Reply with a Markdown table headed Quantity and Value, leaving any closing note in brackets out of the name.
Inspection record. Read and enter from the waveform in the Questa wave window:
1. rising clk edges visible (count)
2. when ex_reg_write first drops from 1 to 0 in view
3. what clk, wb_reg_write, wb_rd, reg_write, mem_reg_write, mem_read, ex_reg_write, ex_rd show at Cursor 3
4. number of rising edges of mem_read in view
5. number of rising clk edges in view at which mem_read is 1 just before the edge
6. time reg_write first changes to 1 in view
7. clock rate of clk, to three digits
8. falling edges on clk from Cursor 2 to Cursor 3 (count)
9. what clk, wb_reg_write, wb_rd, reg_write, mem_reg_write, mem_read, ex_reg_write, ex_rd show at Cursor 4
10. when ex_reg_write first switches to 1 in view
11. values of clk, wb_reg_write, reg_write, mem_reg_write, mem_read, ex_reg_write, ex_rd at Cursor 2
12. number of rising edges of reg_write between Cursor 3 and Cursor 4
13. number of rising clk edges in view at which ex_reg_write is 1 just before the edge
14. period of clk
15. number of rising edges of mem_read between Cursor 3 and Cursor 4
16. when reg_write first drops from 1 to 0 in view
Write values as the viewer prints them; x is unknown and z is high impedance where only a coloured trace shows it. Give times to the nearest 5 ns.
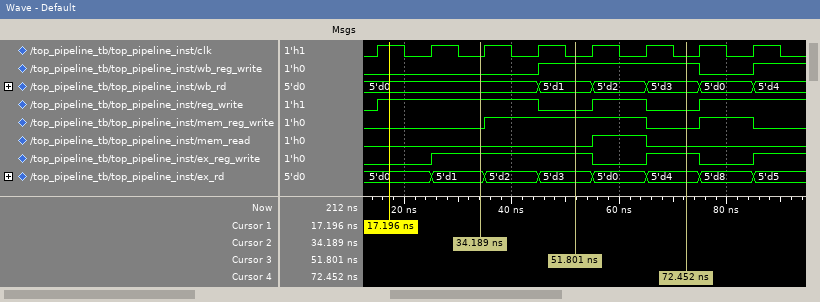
| Quantity | Value |
|---|---|
| rising clk edges visible | 8 |
| when ex_reg_write first drops from 1 to 0 in view | 55 ns |
| what clk, wb_reg_write, wb_rd, reg_write, mem_reg_write, mem_read, ex_reg_write, ex_rd show at Cursor 3 | clk=0, wb_reg_write=1, wb_rd=5'd1, reg_write=0, mem_reg_write=1, mem_read=0, ex_reg_write=1, ex_rd=5'd3 |
| number of rising edges of mem_read in view | 1 |
| number of rising clk edges in view at which mem_read is 1 just before the edge | 1 |
| time reg_write first changes to 1 in view | 15 ns |
| clock rate of clk, to three digits | 100 MHz |
| falling edges on clk from Cursor 2 to Cursor 3 | 2 |
| what clk, wb_reg_write, wb_rd, reg_write, mem_reg_write, mem_read, ex_reg_write, ex_rd show at Cursor 4 | clk=0, wb_reg_write=1, wb_rd=5'd3, reg_write=0, mem_reg_write=0, mem_read=0, ex_reg_write=1, ex_rd=5'd4 |
| when ex_reg_write first switches to 1 in view | 25 ns |
| values of clk, wb_reg_write, reg_write, mem_reg_write, mem_read, ex_reg_write, ex_rd at Cursor 2 | clk=0, wb_reg_write=0, reg_write=1, mem_reg_write=0, mem_read=0, ex_reg_write=1, ex_rd=5'd1 |
| number of rising edges of reg_write between Cursor 3 and Cursor 4 | 1 |
| number of rising clk edges in view at which ex_reg_write is 1 just before the edge | 4 |
| period of clk | 10 ns |
| number of rising edges of mem_read between Cursor 3 and Cursor 4 | 1 |
| when reg_write first drops from 1 to 0 in view | 45 ns |
